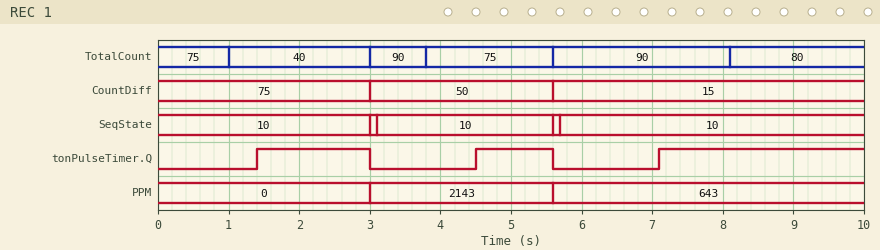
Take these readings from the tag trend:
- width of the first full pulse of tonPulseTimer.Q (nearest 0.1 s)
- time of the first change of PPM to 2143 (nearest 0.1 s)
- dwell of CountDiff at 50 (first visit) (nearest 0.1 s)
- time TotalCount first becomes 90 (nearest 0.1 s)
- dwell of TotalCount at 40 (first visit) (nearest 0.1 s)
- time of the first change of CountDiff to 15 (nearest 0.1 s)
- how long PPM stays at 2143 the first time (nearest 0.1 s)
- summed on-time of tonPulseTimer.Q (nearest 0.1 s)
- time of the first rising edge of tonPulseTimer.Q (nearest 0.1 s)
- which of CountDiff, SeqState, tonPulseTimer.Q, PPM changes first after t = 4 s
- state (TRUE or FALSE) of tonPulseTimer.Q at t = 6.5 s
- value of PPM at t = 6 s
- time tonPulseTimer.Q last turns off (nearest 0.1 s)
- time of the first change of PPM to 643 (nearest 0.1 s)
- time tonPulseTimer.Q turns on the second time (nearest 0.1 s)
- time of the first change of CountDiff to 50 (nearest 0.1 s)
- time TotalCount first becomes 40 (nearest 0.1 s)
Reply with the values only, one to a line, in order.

1.6 s
3.0 s
2.6 s
3.0 s
2.0 s
5.6 s
2.6 s
5.6 s
1.4 s
tonPulseTimer.Q
FALSE
643
5.6 s
5.6 s
4.5 s
3.0 s
1.0 s
